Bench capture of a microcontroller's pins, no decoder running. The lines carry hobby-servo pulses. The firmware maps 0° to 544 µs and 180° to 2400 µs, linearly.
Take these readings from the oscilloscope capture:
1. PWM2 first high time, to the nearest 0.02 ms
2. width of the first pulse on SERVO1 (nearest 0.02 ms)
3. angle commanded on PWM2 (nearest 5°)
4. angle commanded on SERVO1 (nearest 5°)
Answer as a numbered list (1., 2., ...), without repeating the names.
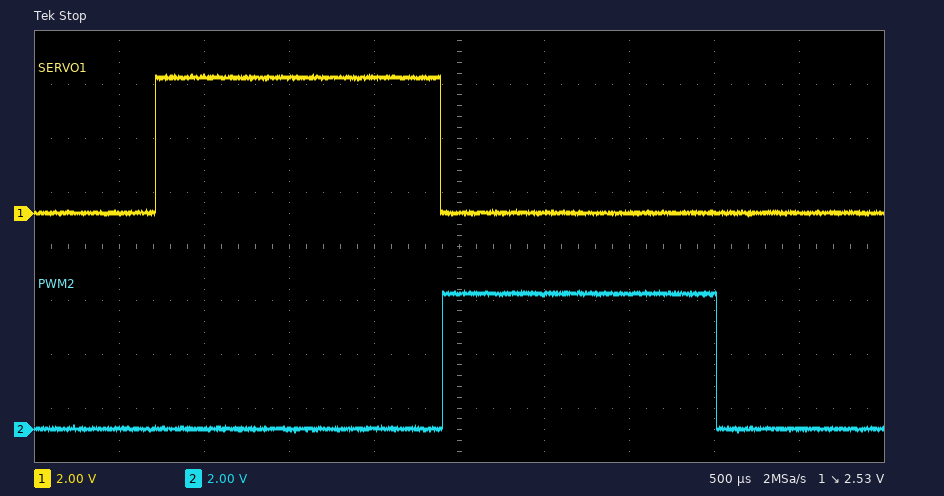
1. 1.62 ms
2. 1.68 ms
3. 105°
4. 110°
